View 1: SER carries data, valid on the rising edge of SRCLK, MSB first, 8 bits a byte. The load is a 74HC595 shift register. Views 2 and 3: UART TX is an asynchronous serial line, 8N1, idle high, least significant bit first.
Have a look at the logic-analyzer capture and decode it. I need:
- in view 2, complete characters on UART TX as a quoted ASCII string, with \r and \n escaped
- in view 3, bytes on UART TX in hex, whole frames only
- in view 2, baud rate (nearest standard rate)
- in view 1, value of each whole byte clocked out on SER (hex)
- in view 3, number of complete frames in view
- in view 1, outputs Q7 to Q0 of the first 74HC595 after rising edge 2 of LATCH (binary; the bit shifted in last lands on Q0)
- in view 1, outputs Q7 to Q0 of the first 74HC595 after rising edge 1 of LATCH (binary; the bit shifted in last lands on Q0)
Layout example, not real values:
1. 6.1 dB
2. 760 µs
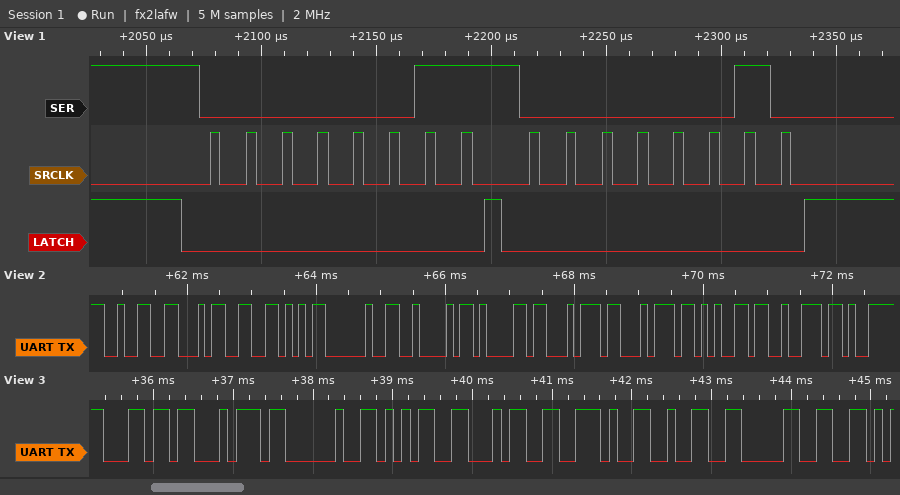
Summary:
1. "24V Batter"
2. 6C 74 20 35 34 2E 32 30
3. 9600 baud
4. 03 02
5. 8
6. 00000010
7. 00000011
